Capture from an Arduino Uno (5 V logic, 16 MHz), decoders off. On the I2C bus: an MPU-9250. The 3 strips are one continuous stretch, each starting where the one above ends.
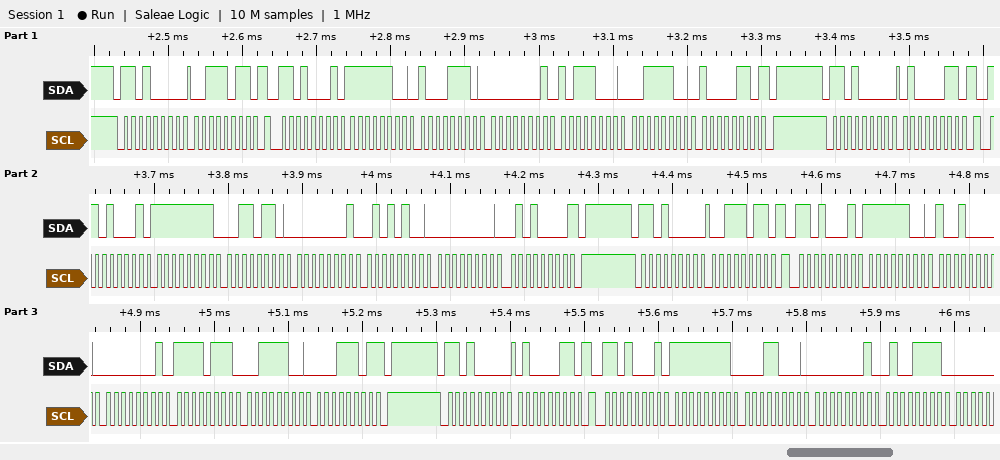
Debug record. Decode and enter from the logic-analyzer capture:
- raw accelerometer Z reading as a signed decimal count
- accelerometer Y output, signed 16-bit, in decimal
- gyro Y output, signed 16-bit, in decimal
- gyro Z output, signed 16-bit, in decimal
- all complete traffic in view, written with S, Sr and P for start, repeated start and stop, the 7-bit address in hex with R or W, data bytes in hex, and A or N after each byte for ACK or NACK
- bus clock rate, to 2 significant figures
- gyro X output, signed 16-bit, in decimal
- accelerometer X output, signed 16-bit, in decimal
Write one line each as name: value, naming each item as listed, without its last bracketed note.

raw accelerometer Z reading as a signed decimal count: 15494
accelerometer Y output, signed 16-bit, in decimal: 440
gyro Y output, signed 16-bit, in decimal: 340
gyro Z output, signed 16-bit, in decimal: 80
all complete traffic in view, written with S, Sr and P for start, repeated start and stop, the 7-bit address in hex with R or W, data bytes in hex, and A or N after each byte for ACK or NACK: S 68W A 3B A Sr 68R A FC A 8E A 01 A B8 A 3C A 86 N P S 68W A 43 A Sr 68R A FF A 36 A 01 A 54 A 00 A 50 N P S 68W A 3B A Sr 68R A FC A 90 A 01 A F7 A 3C A 1D N P S 68W A 43 A Sr 68R A FF A 18 A 01 A 4F A
bus clock rate, to 2 significant figures: 100 kHz
gyro X output, signed 16-bit, in decimal: -202
accelerometer X output, signed 16-bit, in decimal: -882
